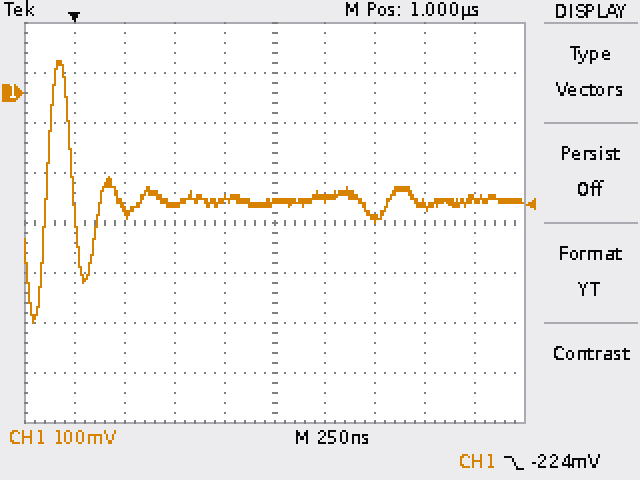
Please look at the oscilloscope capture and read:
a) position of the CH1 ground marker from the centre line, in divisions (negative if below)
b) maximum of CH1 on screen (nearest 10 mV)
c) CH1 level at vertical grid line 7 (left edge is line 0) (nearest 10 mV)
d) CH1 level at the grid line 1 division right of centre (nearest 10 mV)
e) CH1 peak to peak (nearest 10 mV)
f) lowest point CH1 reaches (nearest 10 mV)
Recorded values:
+2.6 div
60 mV
-250 mV
-210 mV
520 mV
-460 mV
